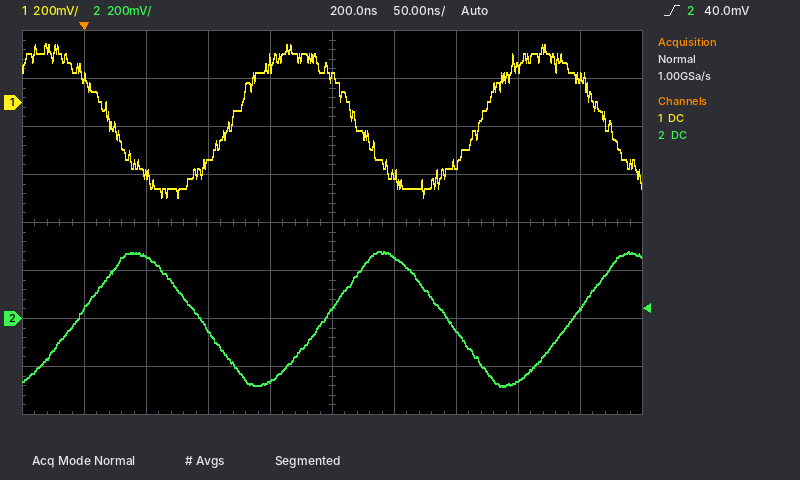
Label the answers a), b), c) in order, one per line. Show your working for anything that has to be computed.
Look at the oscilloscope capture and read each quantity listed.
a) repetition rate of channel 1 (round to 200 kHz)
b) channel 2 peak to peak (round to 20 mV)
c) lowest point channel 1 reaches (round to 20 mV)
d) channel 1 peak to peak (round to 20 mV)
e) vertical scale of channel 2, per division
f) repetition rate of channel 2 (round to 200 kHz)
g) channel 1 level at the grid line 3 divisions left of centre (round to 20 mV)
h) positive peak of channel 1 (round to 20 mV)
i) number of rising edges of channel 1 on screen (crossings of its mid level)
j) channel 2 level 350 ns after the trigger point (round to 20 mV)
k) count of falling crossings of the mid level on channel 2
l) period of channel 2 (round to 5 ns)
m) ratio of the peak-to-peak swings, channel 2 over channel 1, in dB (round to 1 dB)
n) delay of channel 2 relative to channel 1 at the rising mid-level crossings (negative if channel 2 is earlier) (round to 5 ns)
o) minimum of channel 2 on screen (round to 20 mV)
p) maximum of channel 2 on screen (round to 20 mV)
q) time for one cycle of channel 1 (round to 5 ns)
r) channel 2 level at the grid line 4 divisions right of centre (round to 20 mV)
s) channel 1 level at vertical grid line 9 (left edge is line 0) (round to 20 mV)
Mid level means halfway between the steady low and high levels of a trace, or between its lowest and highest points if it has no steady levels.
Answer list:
a) 1 / 200 ns ≈ 5.0 MHz
b) 280 mV − (-280 mV) = 560 mV
c) -400 mV
d) 240 mV − (-400 mV) = 640 mV
e) 200 mV
f) 1 / 200 ns ≈ 5.0 MHz
g) -300 mV
h) 240 mV
i) 2
j) -260 mV
k) 2
l) 200 ns
m) 20 log10(560 mV / 640 mV) ≈ -1 dB
n) +75 ns
o) -280 mV
p) 280 mV
q) 200 ns
r) 40 mV
s) 100 mV
